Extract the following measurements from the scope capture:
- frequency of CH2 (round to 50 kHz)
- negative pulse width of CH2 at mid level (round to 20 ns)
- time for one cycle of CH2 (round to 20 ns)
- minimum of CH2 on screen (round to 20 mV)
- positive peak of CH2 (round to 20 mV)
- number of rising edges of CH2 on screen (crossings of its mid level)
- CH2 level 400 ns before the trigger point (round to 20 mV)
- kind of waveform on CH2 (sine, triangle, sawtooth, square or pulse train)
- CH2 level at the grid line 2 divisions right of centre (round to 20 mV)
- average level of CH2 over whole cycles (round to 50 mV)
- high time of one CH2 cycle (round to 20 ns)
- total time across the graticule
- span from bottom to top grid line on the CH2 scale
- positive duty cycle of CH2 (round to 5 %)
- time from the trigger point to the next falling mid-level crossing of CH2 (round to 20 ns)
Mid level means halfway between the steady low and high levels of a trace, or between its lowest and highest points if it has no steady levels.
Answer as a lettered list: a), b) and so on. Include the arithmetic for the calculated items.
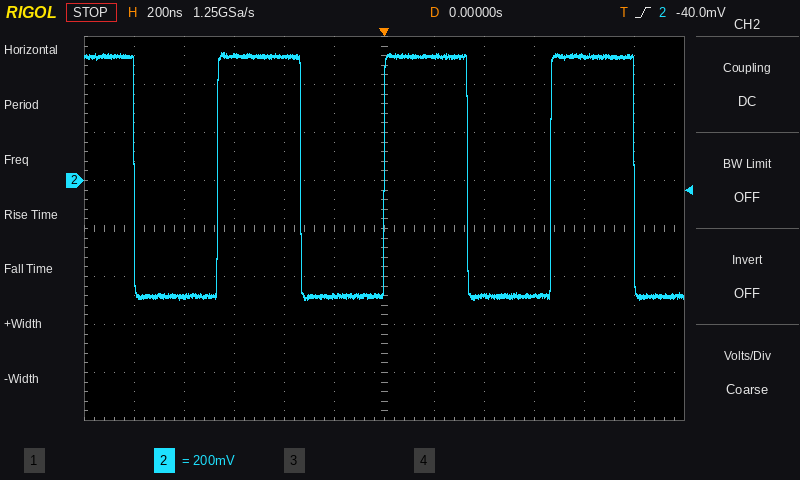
a) 1 / 660 ns ≈ 1.52 MHz, so 1.50 MHz to the nearest 50 kHz
b) 340 ns
c) 660 ns
d) -500 mV
e) 540 mV
f) 3
g) 520 mV
h) square
i) -480 mV
j) -500 mV + 0.5 × (540 mV − (-500 mV)) ≈ 0 mV
k) 340 ns
l) 2.4 µs
m) 1.6 V
n) 340 ns / 660 ns ≈ 51.5 %, so 50 % to the nearest 5 %
o) 340 ns
